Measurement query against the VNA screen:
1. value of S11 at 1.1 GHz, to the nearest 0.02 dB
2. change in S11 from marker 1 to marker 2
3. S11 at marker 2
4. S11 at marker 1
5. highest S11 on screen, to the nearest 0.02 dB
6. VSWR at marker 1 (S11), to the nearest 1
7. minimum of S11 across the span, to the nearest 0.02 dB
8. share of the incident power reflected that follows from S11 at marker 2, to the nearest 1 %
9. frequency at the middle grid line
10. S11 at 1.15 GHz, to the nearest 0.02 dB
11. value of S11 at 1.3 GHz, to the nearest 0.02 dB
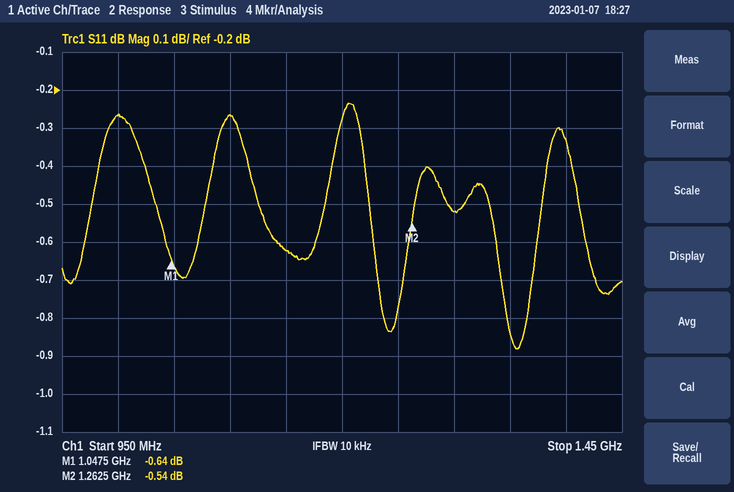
-0.26 dB
0.10 dB
-0.54 dB
-0.64 dB
-0.24 dB
27
-0.88 dB
88 %
1.2 GHz
-0.62 dB
-0.52 dB
